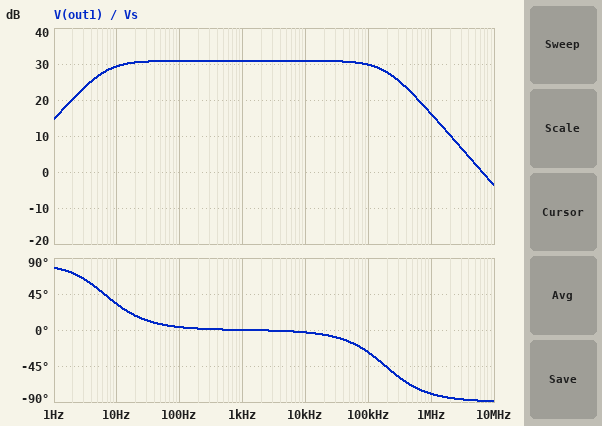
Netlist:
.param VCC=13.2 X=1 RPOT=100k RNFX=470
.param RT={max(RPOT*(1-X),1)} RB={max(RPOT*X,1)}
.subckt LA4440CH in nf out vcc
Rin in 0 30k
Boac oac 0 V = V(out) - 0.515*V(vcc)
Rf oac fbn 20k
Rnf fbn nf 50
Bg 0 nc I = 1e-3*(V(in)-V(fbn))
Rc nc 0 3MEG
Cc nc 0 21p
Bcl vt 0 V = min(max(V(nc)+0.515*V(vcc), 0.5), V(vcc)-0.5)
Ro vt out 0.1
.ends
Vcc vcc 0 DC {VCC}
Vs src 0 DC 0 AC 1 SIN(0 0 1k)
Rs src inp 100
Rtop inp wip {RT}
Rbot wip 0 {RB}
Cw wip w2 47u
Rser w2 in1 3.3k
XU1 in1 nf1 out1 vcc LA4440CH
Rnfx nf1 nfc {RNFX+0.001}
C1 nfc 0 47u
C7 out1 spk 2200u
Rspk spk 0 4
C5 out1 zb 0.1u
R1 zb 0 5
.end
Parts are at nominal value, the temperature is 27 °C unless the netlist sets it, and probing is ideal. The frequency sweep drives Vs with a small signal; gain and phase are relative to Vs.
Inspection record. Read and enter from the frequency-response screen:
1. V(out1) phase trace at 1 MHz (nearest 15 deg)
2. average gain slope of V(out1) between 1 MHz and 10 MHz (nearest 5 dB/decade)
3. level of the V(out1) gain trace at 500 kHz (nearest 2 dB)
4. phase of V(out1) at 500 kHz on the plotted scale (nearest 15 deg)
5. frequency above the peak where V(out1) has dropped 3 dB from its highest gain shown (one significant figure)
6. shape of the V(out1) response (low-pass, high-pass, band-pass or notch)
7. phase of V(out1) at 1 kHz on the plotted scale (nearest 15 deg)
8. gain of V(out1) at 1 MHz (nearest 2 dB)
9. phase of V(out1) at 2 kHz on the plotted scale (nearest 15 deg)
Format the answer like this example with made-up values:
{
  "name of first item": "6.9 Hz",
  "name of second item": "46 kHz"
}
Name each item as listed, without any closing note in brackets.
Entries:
{
  "V(out1) phase trace at 1 MHz": "-75 deg",
  "average gain slope of V(out1) between 1 MHz and 10 MHz": "-20 dB/decade",
  "level of the V(out1) gain trace at 500 kHz": "22 dB",
  "phase of V(out1) at 500 kHz on the plotted scale": "-75 deg",
  "frequency above the peak where V(out1) has dropped 3 dB from its highest gain shown": "200 kHz",
  "shape of the V(out1) response": "band-pass",
  "phase of V(out1) at 1 kHz on the plotted scale": "0 deg",
  "gain of V(out1) at 1 MHz": "16 dB",
  "phase of V(out1) at 2 kHz on the plotted scale": "0 deg"
}
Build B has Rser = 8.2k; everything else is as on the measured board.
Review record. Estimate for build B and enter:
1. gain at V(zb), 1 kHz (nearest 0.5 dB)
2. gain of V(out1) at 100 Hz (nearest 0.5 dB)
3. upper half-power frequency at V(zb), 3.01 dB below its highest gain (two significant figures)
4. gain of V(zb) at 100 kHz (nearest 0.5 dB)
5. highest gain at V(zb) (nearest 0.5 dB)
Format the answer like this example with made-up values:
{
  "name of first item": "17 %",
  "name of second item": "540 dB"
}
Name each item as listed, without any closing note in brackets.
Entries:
{
  "gain at V(zb), 1 kHz": "-20.5 dB",
  "gain of V(out1) at 100 Hz": "29.5 dB",
  "upper half-power frequency at V(zb), 3.01 dB below its highest gain": "600 kHz",
  "gain of V(zb) at 100 kHz": "18.0 dB",
  "highest gain at V(zb)": "21.0 dB"
}
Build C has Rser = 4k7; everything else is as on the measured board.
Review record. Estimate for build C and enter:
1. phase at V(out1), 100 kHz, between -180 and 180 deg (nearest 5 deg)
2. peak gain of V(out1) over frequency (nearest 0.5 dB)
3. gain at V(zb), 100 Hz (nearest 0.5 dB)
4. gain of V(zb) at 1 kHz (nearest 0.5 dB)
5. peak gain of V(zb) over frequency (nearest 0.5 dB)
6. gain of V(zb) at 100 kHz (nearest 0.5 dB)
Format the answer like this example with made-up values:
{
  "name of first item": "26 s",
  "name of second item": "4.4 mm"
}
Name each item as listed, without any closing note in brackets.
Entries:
{
  "phase at V(out1), 100 kHz, between -180 and 180 deg": "-30 deg",
  "peak gain of V(out1) over frequency": "30.5 dB",
  "gain at V(zb), 100 Hz": "-39.5 dB",
  "gain of V(zb) at 1 kHz": "-19.5 dB",
  "peak gain of V(zb) over frequency": "22.0 dB",
  "gain of V(zb) at 100 kHz": "19.0 dB"
}
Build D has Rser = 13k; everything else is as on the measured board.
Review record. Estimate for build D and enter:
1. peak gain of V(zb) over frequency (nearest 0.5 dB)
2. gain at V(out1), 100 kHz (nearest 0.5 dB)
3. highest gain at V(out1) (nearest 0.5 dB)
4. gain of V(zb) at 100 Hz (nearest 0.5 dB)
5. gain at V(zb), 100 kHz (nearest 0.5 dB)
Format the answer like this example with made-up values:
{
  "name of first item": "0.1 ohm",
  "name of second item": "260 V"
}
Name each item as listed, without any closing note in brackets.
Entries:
{
  "peak gain of V(zb) over frequency": "20.0 dB",
  "gain at V(out1), 100 kHz": "27.5 dB",
  "highest gain at V(out1)": "28.5 dB",
  "gain of V(zb) at 100 Hz": "-41.5 dB",
  "gain at V(zb), 100 kHz": "17.0 dB"
}
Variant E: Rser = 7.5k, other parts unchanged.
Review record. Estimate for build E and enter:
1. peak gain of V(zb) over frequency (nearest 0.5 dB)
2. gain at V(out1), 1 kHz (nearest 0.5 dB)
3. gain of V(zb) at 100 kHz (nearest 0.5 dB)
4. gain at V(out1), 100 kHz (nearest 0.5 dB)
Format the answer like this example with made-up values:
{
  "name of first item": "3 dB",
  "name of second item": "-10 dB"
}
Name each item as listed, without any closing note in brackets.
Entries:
{
  "peak gain of V(zb) over frequency": "21.5 dB",
  "gain at V(out1), 1 kHz": "30.0 dB",
  "gain of V(zb) at 100 kHz": "18.5 dB",
  "gain at V(out1), 100 kHz": "29.0 dB"
}
